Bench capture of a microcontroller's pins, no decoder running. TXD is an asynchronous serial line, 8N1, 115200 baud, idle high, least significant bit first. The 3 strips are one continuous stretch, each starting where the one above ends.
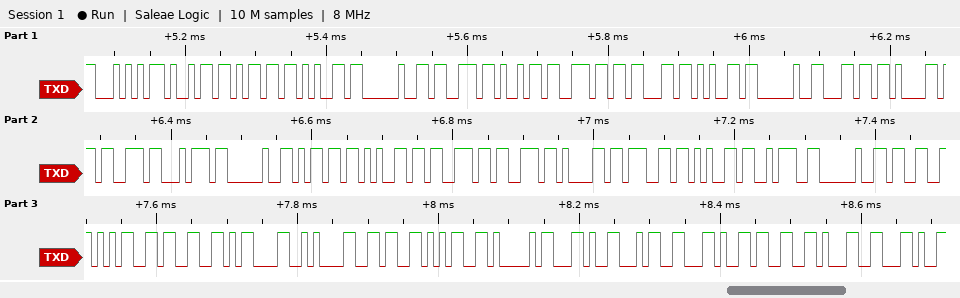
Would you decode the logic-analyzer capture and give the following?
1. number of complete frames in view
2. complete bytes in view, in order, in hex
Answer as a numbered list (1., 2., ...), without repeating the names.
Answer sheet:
1. 39
2. 54 69 6D 65 20 73 69 6E 63 65 20 6C 61 73 74 20 6D 65 73 73 61 67 65 3A 20 33 35 33 0D 0A 36 35 41 2C 34 2C 33 31 2C
